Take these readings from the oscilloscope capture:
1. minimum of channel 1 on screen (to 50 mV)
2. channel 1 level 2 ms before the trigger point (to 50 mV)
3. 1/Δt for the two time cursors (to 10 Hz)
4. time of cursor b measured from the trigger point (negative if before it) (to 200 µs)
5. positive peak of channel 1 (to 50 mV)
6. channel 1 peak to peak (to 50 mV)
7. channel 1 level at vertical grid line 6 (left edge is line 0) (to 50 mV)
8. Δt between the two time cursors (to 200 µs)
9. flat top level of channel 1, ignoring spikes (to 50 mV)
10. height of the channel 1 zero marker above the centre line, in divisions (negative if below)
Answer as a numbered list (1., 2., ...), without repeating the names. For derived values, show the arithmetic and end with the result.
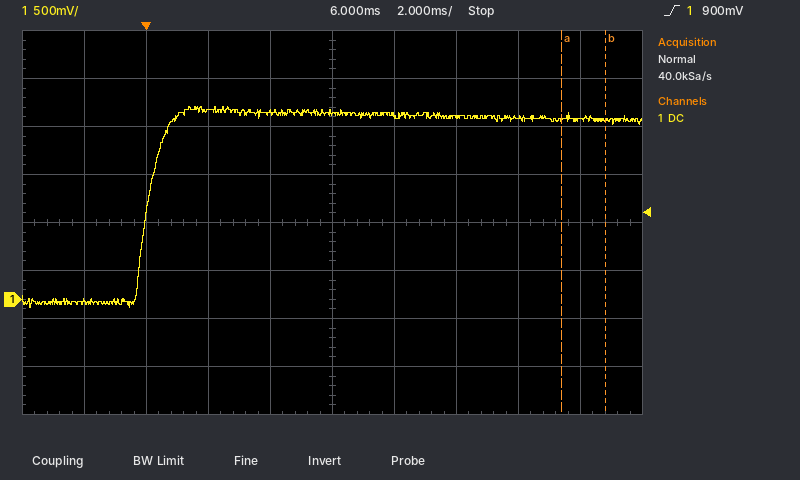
1. -100 mV
2. 0 mV
3. 1 / 1.4 ms ≈ 710 Hz
4. +14.8 ms
5. 2.00 V
6. 2.00 V − (-100 mV) = 2.10 V
7. 1.90 V
8. 1.4 ms
9. 1.90 V
10. -1.6 div
